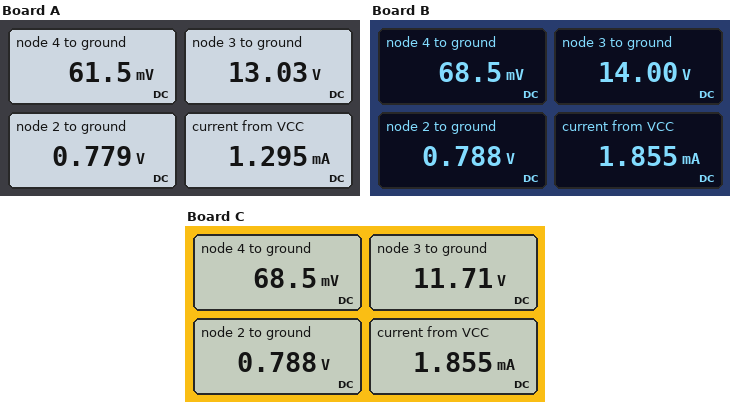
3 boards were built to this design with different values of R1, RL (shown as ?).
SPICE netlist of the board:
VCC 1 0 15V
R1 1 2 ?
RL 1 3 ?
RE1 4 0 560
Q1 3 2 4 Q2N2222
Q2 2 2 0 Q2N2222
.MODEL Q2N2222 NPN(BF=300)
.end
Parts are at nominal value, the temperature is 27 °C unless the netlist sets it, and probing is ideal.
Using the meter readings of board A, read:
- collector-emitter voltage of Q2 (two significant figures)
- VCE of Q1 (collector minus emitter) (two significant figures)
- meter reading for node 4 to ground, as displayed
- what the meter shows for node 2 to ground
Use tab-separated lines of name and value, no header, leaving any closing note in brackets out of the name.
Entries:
collector-emitter voltage of Q2	780 mV
VCE of Q1 (collector minus emitter)	13 V
meter reading for node 4 to ground, as displayed	61.5 mV
what the meter shows for node 2 to ground	0.779 V
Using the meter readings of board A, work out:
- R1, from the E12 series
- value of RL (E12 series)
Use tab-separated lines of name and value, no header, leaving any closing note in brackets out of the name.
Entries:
R1, from the E12 series	12 kΩ
value of RL	18 kΩ
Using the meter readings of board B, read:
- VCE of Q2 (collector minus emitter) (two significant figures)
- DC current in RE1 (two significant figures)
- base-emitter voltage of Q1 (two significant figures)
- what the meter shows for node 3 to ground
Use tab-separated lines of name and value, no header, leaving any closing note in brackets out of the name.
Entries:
VCE of Q2 (collector minus emitter)	790 mV
DC current in RE1	120 µA
base-emitter voltage of Q1	720 mV
what the meter shows for node 3 to ground	14.00 V
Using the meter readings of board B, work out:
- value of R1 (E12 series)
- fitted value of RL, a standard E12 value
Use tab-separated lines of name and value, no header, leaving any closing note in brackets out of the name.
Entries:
value of R1	8.2 kΩ
fitted value of RL, a standard E12 value	8.2 kΩ
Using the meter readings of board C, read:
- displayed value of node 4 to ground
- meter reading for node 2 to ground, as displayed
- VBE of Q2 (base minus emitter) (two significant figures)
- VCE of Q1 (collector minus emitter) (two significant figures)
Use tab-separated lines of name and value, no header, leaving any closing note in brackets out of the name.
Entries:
displayed value of node 4 to ground	68.5 mV
meter reading for node 2 to ground, as displayed	0.788 V
VBE of Q2 (base minus emitter)	790 mV
VCE of Q1 (collector minus emitter)	12 V
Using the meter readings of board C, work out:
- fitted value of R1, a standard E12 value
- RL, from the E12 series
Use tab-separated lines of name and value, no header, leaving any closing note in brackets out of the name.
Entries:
fitted value of R1, a standard E12 value	8.2 kΩ
RL, from the E12 series	27 kΩ
